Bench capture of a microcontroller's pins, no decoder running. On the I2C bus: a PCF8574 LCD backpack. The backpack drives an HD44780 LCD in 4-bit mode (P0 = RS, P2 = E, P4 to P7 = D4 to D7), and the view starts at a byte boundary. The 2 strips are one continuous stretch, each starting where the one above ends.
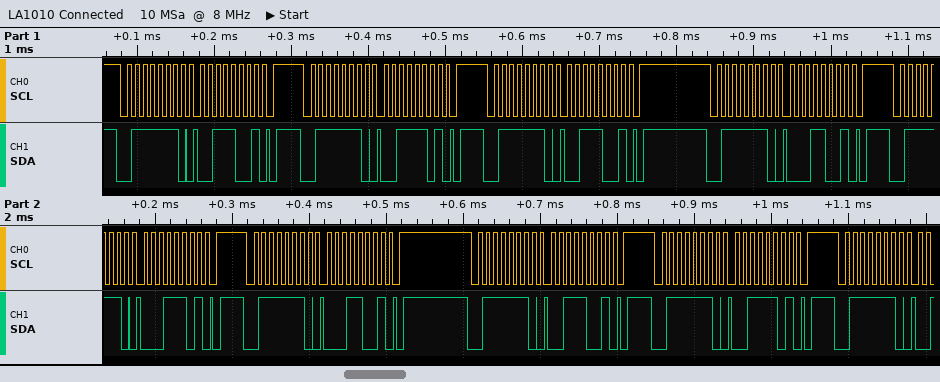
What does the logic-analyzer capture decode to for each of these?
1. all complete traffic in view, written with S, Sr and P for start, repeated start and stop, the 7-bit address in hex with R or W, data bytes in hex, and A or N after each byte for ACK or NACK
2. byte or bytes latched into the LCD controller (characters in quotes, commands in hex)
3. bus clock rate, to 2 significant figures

S 3FW A 39 A P S 3FW A 3D A P S 3FW A 39 A P S 3FW A 19 A P S 3FW A 1D A P S 3FW A 19 A P S 3FW A 39 A P S 3FW A 3D A P S 3FW A
'1'
100 kHz
